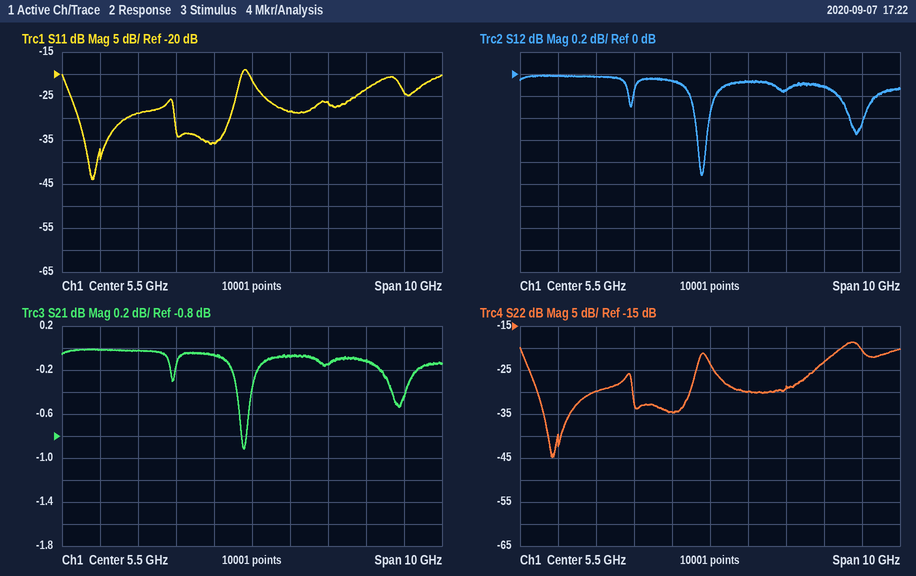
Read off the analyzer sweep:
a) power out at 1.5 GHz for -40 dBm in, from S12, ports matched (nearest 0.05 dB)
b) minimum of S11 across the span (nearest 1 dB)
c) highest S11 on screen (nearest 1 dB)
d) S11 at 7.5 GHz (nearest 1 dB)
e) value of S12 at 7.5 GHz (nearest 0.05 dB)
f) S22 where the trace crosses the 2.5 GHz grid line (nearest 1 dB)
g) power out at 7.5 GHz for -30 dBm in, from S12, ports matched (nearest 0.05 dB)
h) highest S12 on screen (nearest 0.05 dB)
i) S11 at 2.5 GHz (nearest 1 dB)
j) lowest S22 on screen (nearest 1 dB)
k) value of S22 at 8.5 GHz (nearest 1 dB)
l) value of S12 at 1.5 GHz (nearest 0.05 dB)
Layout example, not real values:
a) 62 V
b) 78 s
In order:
a) -40.00 dBm
b) -44 dB
c) -19 dB
d) -26 dB
e) -0.15 dB
f) -30 dB
g) -30.15 dBm
h) 0.00 dB
i) -29 dB
j) -45 dB
k) -23 dB
l) 0.00 dB
